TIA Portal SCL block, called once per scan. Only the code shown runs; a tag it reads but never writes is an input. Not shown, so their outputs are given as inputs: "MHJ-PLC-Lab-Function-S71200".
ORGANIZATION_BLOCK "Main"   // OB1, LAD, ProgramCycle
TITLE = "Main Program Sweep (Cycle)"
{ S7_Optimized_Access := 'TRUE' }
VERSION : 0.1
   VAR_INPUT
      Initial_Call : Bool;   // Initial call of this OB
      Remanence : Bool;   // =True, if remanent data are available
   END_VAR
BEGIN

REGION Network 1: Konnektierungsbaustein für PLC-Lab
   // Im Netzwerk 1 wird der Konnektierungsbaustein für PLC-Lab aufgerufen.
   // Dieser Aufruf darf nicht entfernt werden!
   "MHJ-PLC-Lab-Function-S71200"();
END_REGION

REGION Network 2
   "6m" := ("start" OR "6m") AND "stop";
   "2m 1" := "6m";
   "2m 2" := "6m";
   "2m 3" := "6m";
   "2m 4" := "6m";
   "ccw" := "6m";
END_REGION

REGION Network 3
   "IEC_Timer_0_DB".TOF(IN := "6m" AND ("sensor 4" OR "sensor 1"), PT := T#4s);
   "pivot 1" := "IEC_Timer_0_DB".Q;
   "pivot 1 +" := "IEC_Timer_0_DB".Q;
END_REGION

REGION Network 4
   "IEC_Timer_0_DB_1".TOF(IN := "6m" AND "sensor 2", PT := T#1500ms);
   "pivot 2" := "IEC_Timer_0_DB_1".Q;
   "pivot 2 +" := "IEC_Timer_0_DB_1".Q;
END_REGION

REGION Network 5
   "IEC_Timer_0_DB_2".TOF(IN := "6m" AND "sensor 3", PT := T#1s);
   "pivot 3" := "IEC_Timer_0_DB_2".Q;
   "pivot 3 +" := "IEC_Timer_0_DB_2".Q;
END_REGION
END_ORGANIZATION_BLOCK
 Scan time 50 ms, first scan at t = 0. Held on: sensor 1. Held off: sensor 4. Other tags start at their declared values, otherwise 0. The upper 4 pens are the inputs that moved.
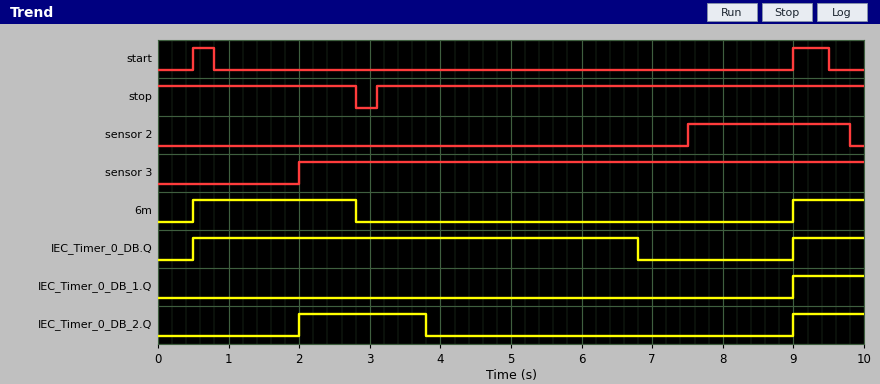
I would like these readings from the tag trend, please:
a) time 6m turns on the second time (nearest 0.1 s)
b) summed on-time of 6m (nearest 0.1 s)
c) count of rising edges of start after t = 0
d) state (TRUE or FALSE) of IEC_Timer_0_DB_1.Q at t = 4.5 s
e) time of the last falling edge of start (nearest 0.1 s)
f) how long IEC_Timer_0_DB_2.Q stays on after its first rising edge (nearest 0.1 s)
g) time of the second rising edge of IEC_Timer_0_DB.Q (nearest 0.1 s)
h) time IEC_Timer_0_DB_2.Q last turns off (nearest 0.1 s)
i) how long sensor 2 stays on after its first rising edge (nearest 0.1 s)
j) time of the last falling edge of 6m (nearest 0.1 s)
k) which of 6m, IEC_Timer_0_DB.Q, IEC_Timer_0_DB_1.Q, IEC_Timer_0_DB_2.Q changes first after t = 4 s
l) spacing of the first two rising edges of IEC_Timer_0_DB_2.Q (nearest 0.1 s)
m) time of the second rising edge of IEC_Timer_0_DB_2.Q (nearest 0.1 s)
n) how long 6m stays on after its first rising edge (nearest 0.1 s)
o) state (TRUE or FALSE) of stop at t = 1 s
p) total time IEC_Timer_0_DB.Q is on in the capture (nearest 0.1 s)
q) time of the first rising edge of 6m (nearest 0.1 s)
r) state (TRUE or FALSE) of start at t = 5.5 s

9.0 s
3.3 s
2
FALSE
9.5 s
1.8 s
9.0 s
3.8 s
2.3 s
2.8 s
IEC_Timer_0_DB.Q
7.0 s
9.0 s
2.3 s
TRUE
7.3 s
0.5 s
FALSE
